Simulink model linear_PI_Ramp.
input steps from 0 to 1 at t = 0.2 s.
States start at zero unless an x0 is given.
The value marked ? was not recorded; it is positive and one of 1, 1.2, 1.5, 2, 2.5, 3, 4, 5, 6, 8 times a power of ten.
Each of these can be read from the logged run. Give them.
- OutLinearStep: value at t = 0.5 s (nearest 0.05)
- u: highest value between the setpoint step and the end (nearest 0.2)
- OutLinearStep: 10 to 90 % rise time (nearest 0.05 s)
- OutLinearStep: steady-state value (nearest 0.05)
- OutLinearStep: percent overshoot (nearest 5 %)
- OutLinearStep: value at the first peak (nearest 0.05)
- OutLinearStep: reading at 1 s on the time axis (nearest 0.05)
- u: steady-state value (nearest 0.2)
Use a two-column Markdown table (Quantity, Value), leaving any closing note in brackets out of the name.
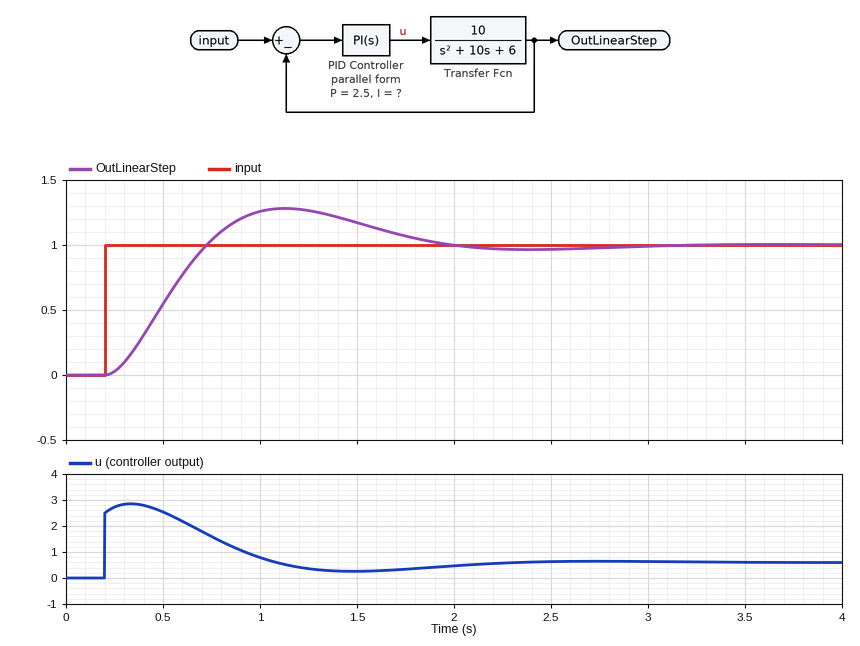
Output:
| Quantity | Value |
|---|---|
| OutLinearStep: value at t = 0.5 s | 0.55 |
| u: highest value between the setpoint step and the end | 2.8 |
| OutLinearStep: 10 to 90 % rise time | 0.35 s |
| OutLinearStep: steady-state value | 1.00 |
| OutLinearStep: percent overshoot | 30 % |
| OutLinearStep: value at the first peak | 1.30 |
| OutLinearStep: reading at 1 s on the time axis | 1.25 |
| u: steady-state value | 0.6 |
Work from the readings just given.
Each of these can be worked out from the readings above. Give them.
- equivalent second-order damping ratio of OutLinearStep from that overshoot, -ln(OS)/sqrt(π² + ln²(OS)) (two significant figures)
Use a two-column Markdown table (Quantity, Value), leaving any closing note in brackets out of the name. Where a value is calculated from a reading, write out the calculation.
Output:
| Quantity | Value |
|---|---|
| equivalent second-order damping ratio of OutLinearStep from that overshoot, -ln(OS)/sqrt(π² + ln²(OS)) | ln(0.3) = -1.204; 1.204 / sqrt(9.870 + 1.450) = 0.36 |
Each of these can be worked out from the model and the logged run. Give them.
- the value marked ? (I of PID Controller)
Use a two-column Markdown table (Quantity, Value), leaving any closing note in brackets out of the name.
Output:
| Quantity | Value |
|---|---|
| the value marked ? | 6 |
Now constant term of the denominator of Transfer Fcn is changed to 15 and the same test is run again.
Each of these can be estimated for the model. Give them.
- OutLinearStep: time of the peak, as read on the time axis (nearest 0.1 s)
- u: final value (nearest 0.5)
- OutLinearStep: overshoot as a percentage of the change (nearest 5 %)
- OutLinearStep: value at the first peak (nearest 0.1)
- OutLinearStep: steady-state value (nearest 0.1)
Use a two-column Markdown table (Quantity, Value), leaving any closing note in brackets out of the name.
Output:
| Quantity | Value |
|---|---|
| OutLinearStep: time of the peak, as read on the time axis | 1.1 s |
| u: final value | 1.5 |
| OutLinearStep: overshoot as a percentage of the change | 10 % |
| OutLinearStep: value at the first peak | 1.1 |
| OutLinearStep: steady-state value | 1.0 |
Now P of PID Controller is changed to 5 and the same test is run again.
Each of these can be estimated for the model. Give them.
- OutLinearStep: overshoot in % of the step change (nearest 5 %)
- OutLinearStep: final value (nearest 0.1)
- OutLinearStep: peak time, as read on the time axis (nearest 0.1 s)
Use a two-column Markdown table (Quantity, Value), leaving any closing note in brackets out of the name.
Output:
| Quantity | Value |
|---|---|
| OutLinearStep: overshoot in % of the step change | 15 % |
| OutLinearStep: final value | 1.0 |
| OutLinearStep: peak time, as read on the time axis | 0.8 s |
